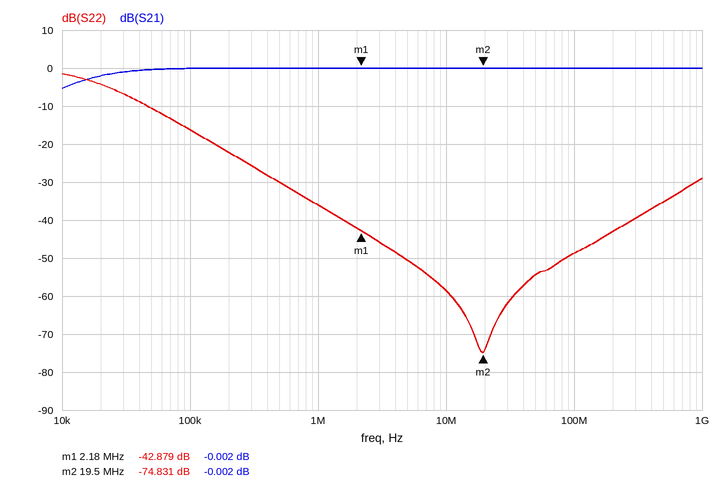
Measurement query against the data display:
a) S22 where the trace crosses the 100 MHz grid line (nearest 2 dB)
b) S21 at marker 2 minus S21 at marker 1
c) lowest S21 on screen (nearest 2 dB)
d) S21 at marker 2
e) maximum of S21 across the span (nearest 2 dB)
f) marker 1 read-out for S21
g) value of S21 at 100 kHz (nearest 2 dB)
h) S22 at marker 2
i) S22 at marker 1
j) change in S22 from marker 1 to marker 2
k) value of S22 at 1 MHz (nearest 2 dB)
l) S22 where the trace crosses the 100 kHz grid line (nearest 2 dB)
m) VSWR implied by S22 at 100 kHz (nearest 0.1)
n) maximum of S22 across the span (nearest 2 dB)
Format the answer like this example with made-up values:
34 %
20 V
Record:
-48 dB
0.000 dB
-6 dB
-0.002 dB
0 dB
-0.002 dB
0 dB
-74.831 dB
-42.879 dB
-31.952 dB
-36 dB
-16 dB
1.4
-2 dB
